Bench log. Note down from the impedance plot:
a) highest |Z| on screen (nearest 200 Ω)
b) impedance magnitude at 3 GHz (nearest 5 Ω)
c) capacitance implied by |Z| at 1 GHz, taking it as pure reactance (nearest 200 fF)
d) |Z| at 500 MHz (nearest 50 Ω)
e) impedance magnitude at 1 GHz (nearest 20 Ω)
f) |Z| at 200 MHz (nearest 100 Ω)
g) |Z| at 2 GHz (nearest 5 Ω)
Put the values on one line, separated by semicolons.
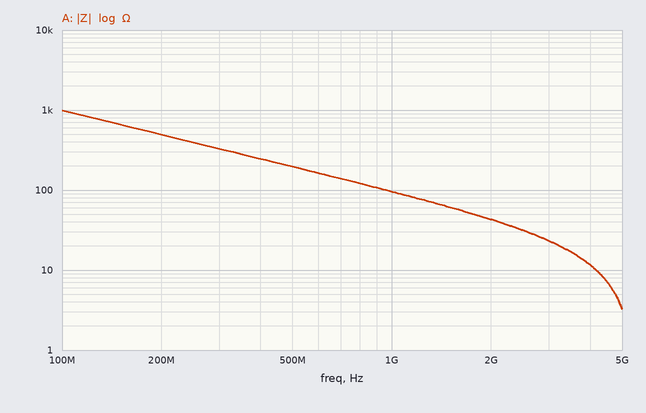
1.0 kΩ; 25 Ω; 1.6 pF; 200 Ω; 100 Ω; 500 Ω; 45 Ω
